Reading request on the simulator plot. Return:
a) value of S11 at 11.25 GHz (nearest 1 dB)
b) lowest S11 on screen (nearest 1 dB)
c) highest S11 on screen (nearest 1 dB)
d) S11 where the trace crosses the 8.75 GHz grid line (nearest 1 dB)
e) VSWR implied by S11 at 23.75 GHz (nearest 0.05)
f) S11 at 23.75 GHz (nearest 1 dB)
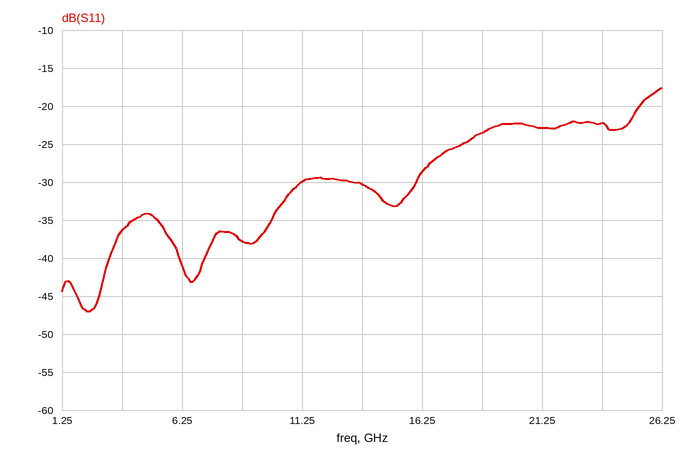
-30 dB
-47 dB
-18 dB
-38 dB
1.15
-22 dB
